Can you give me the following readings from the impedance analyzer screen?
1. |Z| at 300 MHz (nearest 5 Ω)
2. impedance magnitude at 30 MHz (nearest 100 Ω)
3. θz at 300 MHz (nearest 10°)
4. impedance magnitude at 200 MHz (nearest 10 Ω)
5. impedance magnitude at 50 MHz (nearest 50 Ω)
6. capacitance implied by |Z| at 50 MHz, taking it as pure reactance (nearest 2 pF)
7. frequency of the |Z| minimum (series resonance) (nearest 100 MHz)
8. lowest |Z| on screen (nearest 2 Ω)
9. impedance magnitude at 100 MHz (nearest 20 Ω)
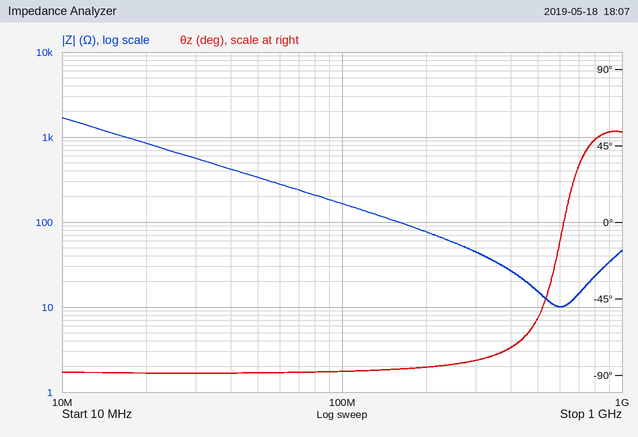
45 Ω
600 Ω
-80°
80 Ω
350 Ω
10 pF
600 MHz
10 Ω
160 Ω
